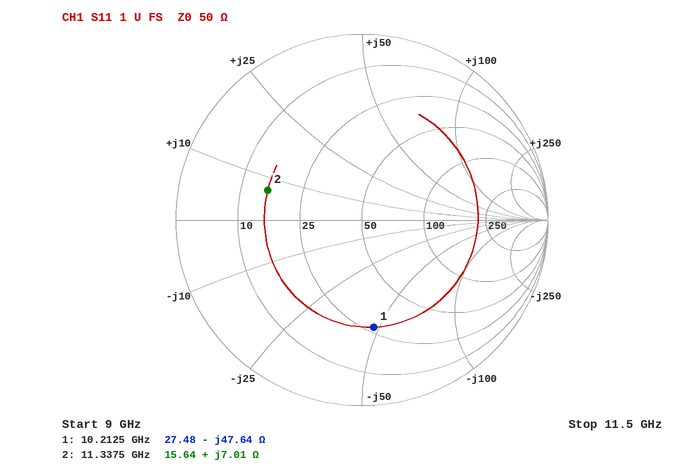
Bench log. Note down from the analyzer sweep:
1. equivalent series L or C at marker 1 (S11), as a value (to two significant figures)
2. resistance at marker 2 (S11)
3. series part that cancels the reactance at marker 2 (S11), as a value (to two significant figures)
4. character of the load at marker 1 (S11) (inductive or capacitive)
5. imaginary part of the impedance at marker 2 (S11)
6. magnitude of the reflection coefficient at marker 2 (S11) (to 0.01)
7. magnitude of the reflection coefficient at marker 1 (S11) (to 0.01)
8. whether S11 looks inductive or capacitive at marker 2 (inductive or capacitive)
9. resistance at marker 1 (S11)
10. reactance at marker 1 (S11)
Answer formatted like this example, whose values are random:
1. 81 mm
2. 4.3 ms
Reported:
1. 330 fF
2. 15.64 Ω
3. 2.0 pF
4. capacitive
5. +7.01 Ω
6. 0.53
7. 0.58
8. inductive
9. 27.48 Ω
10. -47.64 Ω
